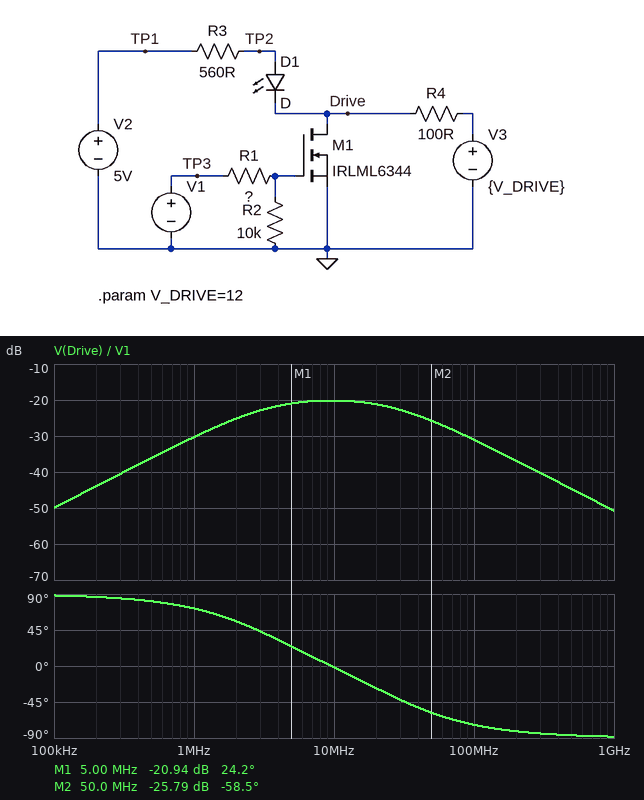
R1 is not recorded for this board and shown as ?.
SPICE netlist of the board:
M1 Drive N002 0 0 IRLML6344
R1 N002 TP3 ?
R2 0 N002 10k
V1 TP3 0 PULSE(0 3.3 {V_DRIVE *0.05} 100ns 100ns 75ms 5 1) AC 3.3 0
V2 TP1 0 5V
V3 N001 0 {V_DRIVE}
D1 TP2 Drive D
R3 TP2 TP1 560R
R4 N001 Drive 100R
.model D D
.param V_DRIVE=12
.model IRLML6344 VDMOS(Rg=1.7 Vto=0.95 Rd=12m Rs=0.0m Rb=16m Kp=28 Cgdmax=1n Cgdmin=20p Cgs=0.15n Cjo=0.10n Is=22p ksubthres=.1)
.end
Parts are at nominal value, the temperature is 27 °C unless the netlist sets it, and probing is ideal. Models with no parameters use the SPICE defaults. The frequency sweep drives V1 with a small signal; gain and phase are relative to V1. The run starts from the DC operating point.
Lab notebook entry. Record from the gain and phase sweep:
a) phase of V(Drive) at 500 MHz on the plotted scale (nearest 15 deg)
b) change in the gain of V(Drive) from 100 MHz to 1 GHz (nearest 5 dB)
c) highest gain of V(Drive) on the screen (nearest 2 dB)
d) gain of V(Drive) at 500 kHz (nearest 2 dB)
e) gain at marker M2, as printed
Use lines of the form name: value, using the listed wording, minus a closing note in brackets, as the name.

phase of V(Drive) at 500 MHz on the plotted scale: -90 deg
change in the gain of V(Drive) from 100 MHz to 1 GHz: -20 dB
highest gain of V(Drive) on the screen: -20 dB
gain of V(Drive) at 500 kHz: -36 dB
gain at marker M2, as printed: -25.79 dB
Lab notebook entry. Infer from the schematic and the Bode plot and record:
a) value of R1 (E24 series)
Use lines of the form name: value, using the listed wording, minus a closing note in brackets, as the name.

value of R1: 220 Ω
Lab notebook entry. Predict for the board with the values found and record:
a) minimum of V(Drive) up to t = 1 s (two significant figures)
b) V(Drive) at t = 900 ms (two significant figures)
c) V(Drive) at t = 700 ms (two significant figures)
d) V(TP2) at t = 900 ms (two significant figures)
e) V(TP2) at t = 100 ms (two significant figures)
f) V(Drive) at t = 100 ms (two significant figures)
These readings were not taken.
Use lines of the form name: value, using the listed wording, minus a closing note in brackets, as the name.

minimum of V(Drive) up to t = 1 s: 3.5 mV
V(Drive) at t = 900 ms: 12 V
V(Drive) at t = 700 ms: 12 V
V(TP2) at t = 900 ms: 5.0 V
V(TP2) at t = 100 ms: 5.0 V
V(Drive) at t = 100 ms: 12 V
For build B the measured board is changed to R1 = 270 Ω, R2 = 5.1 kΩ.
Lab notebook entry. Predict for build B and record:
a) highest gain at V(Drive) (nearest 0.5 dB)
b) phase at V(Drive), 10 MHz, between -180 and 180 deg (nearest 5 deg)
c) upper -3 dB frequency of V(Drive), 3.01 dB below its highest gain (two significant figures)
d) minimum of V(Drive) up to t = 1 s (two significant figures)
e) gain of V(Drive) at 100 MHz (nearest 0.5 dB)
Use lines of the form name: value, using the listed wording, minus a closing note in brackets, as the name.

highest gain at V(Drive): -21.5 dB
phase at V(Drive), 10 MHz, between -180 and 180 deg: -5 deg
upper -3 dB frequency of V(Drive), 3.01 dB below its highest gain: 31 MHz
minimum of V(Drive) up to t = 1 s: 3.6 mV
gain of V(Drive) at 100 MHz: -33.0 dB
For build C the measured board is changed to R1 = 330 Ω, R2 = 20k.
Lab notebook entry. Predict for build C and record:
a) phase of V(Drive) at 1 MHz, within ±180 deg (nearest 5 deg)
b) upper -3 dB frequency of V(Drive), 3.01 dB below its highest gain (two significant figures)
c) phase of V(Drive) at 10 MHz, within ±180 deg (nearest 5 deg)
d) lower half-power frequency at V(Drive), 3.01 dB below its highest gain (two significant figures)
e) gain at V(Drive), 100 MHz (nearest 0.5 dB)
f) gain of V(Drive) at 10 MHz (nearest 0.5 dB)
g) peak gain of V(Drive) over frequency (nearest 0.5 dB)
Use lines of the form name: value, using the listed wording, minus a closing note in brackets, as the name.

phase of V(Drive) at 1 MHz, within ±180 deg: 65 deg
upper -3 dB frequency of V(Drive), 3.01 dB below its highest gain: 30 MHz
phase of V(Drive) at 10 MHz, within ±180 deg: -10 deg
lower half-power frequency at V(Drive), 3.01 dB below its highest gain: 2.0 MHz
gain at V(Drive), 100 MHz: -34.5 dB
gain of V(Drive) at 10 MHz: -23.5 dB
peak gain of V(Drive) over frequency: -23.0 dB
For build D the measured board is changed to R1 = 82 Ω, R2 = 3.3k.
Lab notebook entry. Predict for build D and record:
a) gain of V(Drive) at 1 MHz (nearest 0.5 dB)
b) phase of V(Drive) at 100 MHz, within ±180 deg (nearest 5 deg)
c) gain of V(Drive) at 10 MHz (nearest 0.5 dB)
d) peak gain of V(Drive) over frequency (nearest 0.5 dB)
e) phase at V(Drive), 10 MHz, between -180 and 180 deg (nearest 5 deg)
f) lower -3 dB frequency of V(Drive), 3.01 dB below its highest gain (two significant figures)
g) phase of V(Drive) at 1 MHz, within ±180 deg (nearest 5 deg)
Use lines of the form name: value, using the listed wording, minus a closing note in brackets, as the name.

gain of V(Drive) at 1 MHz: -30.0 dB
phase of V(Drive) at 100 MHz, within ±180 deg: -70 deg
gain of V(Drive) at 10 MHz: -14.0 dB
peak gain of V(Drive) over frequency: -13.5 dB
phase at V(Drive), 10 MHz, between -180 and 180 deg: 20 deg
lower -3 dB frequency of V(Drive), 3.01 dB below its highest gain: 5.7 MHz
phase of V(Drive) at 1 MHz, within ±180 deg: 80 deg
